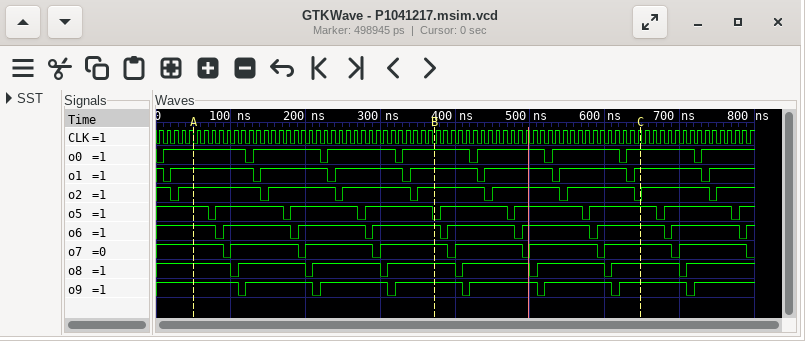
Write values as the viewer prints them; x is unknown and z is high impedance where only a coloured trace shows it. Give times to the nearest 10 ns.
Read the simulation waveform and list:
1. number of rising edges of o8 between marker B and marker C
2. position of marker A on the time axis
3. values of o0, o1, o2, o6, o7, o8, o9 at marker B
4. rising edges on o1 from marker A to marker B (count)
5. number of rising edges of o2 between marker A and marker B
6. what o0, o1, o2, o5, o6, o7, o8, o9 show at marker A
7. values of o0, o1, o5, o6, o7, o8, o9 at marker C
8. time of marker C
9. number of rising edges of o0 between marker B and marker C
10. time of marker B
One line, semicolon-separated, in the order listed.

3; 50 ns; o0=1, o1=1, o2=1, o6=1, o7=1, o8=1, o9=1; 3; 3; o0=1, o1=1, o2=1, o5=1, o6=1, o7=1, o8=1, o9=1; o0=1, o1=1, o5=1, o6=1, o7=1, o8=1, o9=1; 650 ns; 3; 370 ns
